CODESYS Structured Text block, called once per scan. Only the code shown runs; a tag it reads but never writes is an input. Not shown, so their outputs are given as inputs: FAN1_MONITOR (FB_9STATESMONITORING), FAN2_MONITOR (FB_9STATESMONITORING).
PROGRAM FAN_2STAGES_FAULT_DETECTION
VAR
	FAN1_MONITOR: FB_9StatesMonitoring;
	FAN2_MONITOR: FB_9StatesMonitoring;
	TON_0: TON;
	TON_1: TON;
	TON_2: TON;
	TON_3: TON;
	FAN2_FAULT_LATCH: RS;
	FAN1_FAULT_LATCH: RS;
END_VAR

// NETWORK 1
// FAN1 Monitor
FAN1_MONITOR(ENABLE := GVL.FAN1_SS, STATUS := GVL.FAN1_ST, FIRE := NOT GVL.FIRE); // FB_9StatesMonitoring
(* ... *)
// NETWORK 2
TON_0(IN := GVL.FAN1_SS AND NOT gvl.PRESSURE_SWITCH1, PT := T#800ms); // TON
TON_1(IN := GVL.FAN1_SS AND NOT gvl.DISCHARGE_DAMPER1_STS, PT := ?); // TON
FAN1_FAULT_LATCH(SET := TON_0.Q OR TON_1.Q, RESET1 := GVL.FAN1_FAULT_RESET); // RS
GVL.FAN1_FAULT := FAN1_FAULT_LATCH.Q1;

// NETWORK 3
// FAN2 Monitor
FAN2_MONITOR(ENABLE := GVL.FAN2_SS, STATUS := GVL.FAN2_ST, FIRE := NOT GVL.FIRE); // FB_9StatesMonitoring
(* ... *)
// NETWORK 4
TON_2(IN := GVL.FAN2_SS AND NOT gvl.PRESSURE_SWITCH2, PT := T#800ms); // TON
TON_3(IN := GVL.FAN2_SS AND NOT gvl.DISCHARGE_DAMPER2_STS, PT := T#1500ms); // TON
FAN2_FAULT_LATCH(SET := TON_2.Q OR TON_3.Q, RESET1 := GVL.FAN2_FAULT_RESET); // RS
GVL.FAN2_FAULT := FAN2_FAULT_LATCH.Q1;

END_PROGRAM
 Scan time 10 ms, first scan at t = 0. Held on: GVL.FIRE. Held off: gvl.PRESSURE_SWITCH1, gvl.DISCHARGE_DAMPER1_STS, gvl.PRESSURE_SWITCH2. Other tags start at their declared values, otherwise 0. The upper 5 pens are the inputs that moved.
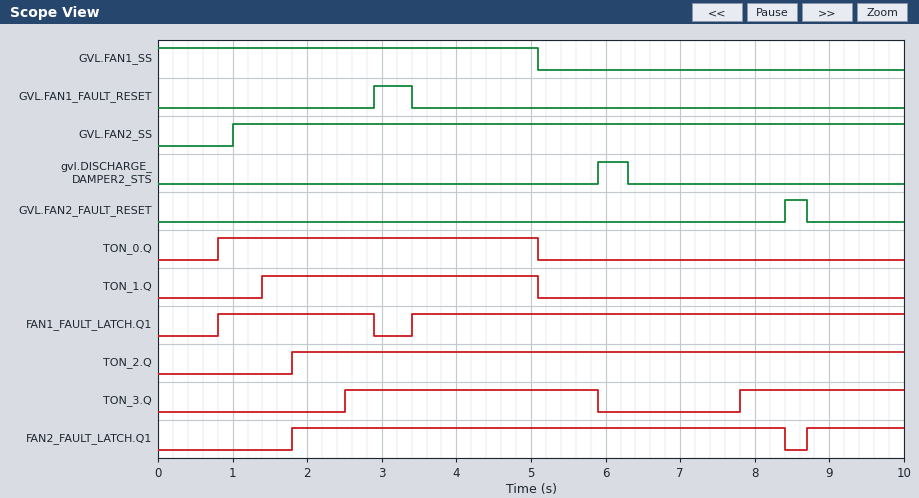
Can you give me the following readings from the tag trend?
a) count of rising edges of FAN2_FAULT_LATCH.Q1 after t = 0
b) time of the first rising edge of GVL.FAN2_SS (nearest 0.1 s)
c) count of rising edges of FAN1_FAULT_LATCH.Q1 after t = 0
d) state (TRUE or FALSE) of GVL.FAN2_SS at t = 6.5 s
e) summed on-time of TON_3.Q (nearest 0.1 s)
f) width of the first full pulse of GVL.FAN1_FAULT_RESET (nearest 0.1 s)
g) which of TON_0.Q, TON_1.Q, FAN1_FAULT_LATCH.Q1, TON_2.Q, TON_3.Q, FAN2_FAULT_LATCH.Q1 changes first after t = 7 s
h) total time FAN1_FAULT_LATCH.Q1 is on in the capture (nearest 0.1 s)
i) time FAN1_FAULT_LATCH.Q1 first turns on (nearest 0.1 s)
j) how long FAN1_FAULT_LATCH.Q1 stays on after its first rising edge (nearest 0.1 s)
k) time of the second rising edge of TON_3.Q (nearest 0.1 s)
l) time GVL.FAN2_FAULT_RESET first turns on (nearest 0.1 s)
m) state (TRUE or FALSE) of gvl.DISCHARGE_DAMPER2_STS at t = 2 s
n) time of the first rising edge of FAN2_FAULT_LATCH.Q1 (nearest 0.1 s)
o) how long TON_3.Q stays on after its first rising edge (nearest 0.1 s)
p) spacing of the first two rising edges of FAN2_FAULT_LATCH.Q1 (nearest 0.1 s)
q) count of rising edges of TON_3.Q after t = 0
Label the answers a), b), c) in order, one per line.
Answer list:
a) 2
b) 1.0 s
c) 2
d) TRUE
e) 5.6 s
f) 0.5 s
g) TON_3.Q
h) 8.7 s
i) 0.8 s
j) 2.1 s
k) 7.8 s
l) 8.4 s
m) FALSE
n) 1.8 s
o) 3.4 s
p) 6.9 s
q) 2
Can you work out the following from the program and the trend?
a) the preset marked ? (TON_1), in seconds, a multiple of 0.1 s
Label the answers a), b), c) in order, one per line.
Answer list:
a) 1.4 s
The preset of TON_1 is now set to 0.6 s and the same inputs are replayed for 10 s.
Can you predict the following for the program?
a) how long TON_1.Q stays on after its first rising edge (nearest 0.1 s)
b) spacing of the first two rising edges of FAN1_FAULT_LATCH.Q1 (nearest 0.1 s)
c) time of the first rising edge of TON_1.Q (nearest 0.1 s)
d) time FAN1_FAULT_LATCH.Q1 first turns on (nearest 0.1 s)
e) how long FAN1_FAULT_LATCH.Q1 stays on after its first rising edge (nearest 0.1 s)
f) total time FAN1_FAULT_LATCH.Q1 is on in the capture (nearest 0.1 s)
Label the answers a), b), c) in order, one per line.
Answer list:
a) 4.5 s
b) 2.8 s
c) 0.6 s
d) 0.6 s
e) 2.3 s
f) 8.9 s
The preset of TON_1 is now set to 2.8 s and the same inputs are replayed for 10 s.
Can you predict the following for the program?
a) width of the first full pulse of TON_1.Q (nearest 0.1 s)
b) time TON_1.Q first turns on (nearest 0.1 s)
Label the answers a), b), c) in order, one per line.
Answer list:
a) 2.3 s
b) 2.8 s
